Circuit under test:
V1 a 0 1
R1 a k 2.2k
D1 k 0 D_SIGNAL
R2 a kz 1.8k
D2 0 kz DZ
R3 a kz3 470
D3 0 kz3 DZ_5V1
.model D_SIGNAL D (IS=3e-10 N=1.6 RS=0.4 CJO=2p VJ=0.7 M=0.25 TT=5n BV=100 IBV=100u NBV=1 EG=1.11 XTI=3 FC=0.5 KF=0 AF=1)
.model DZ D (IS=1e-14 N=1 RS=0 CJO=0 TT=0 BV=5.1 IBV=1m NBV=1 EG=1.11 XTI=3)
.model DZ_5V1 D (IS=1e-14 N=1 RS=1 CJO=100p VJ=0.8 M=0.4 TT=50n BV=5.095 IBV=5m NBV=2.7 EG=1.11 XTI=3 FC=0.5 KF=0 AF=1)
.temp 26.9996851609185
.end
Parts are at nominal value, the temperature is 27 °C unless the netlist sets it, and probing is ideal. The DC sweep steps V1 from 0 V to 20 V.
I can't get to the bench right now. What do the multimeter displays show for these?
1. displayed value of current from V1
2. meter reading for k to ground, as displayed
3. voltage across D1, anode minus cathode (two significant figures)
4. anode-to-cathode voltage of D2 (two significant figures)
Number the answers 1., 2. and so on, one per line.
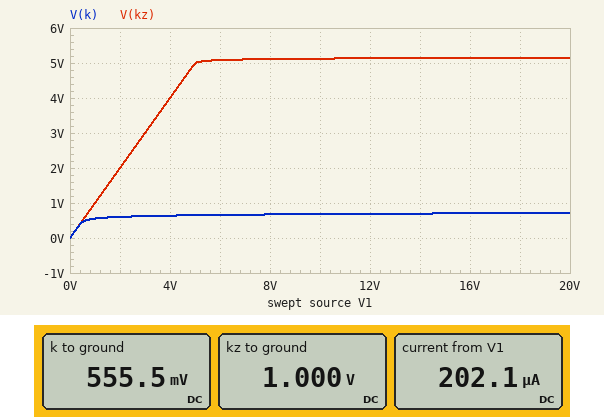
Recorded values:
1. 202.1 µA
2. 555.5 mV
3. 560 mV
4. -1.0 V
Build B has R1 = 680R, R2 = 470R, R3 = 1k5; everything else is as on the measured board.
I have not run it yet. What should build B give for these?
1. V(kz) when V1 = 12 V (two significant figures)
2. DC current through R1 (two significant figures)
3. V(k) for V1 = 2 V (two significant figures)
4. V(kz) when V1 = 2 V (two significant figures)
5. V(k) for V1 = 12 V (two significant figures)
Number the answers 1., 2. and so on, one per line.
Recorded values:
1. 5.2 V
2. 590 µA
3. 650 mV
4. 2.0 V
5. 740 mV
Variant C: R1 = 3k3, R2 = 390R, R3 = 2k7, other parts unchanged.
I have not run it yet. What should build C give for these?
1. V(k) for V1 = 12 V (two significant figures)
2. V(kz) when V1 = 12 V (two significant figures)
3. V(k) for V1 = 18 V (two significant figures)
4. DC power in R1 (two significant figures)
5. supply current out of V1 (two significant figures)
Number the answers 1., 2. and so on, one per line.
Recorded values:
1. 670 mV
2. 5.2 V
3. 690 mV
4. 64 µW
5. 140 µA
